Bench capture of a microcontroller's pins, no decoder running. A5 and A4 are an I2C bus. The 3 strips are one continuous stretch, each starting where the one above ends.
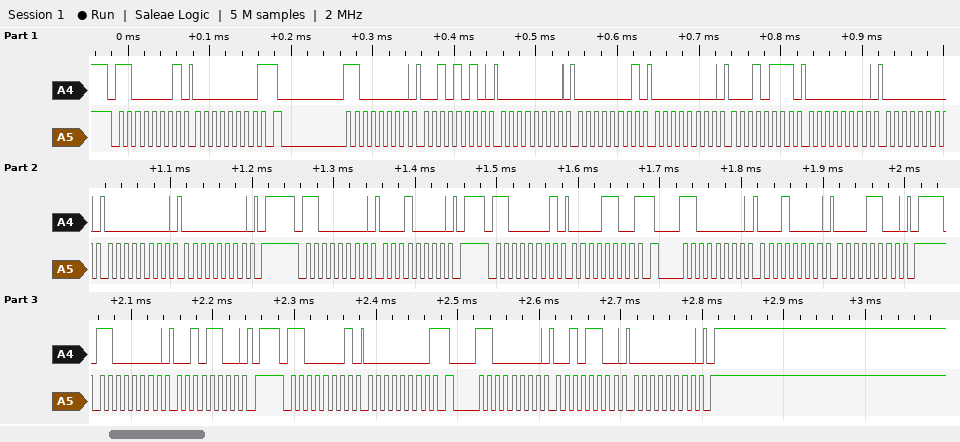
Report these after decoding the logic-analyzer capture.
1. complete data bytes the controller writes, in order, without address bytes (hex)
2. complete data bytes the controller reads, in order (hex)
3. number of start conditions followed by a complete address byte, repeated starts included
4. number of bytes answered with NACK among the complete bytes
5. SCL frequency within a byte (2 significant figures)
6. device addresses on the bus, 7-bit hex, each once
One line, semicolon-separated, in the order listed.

2A 00 01 00 17 00 00 00 00 10 10 0C 2C 2C 00; 00 0C 00; 8; 3; 100 kHz; 0x60
